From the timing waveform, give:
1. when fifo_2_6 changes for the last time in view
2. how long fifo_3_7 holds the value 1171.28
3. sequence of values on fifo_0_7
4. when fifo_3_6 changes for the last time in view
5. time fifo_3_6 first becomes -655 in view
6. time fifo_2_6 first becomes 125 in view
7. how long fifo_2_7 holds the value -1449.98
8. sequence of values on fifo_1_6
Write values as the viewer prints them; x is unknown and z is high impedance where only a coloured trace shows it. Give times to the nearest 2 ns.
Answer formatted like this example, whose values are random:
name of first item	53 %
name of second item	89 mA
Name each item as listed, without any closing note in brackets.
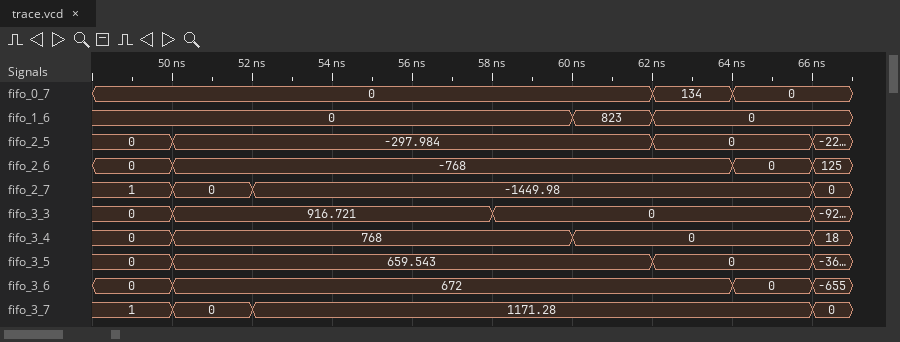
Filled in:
when fifo_2_6 changes for the last time in view	66 ns
how long fifo_3_7 holds the value 1171.28	14 ns
sequence of values on fifo_0_7	0, 134, 0
when fifo_3_6 changes for the last time in view	66 ns
time fifo_3_6 first becomes -655 in view	66 ns
time fifo_2_6 first becomes 125 in view	66 ns
how long fifo_2_7 holds the value -1449.98	14 ns
sequence of values on fifo_1_6	0, 823, 0
